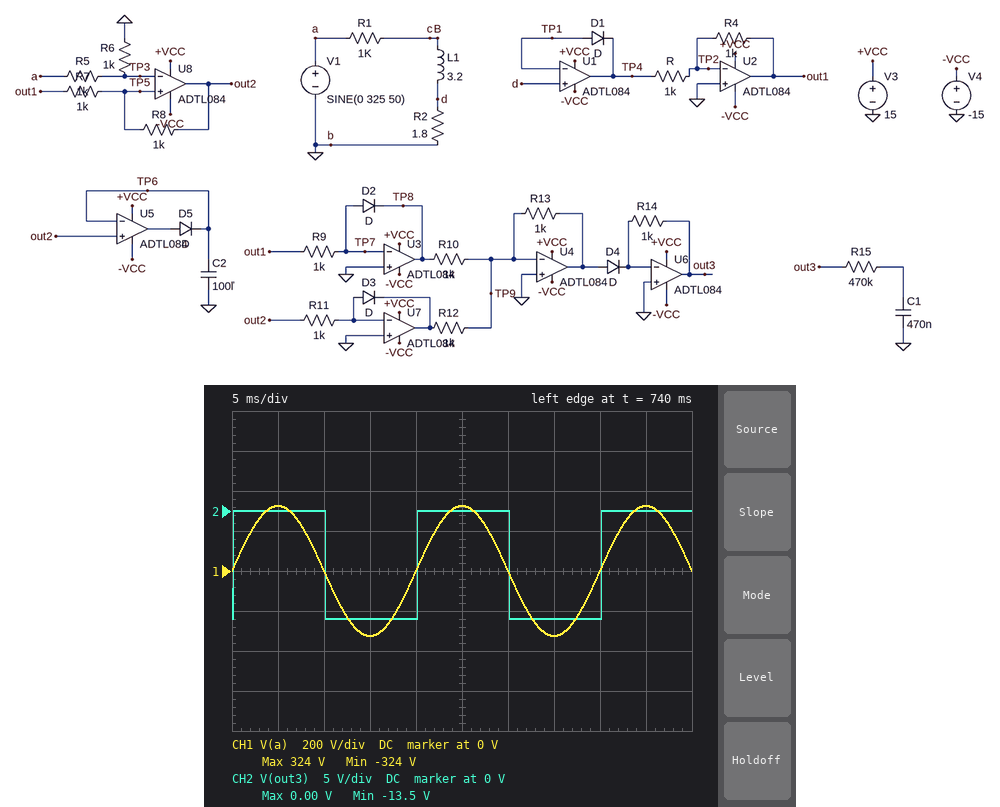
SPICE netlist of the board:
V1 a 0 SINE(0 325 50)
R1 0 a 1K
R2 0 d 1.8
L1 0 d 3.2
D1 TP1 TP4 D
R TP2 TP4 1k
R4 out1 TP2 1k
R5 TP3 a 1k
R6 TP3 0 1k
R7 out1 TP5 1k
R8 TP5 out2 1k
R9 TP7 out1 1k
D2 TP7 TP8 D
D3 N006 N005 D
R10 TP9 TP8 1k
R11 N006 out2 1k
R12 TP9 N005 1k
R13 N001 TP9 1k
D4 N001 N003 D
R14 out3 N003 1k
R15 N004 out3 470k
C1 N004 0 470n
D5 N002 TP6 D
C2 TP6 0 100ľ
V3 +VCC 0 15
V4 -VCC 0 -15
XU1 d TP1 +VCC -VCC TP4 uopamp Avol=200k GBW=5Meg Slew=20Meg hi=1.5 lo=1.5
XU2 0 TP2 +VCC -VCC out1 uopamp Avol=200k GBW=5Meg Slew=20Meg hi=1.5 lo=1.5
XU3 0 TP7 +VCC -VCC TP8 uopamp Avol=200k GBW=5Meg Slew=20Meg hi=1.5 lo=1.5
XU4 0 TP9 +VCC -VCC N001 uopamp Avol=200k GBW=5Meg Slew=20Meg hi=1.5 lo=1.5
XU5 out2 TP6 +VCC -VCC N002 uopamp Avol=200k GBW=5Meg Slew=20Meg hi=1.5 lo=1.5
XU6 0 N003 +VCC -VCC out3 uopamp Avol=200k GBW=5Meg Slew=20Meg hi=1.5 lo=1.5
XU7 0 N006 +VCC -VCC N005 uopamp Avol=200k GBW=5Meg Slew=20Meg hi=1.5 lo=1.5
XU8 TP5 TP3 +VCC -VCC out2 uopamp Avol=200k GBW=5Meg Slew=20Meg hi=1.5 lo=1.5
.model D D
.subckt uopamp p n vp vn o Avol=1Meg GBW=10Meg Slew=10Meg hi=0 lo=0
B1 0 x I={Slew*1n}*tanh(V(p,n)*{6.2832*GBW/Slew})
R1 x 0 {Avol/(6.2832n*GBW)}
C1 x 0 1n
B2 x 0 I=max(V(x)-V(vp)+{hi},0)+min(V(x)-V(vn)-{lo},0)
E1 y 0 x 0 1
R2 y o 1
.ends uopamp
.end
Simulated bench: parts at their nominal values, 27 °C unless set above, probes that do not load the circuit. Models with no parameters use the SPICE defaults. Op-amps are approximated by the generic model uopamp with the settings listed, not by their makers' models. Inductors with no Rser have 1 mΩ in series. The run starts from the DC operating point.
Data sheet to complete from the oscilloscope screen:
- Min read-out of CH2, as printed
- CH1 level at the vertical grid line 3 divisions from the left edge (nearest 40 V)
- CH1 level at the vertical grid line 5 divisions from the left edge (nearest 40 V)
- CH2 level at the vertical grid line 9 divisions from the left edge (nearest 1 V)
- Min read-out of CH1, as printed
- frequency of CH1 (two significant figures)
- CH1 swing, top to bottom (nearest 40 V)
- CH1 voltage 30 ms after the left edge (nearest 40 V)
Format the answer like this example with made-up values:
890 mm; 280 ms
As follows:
-13.5 V; -320 V; 320 V; 0 V; -324 V; 50 Hz; 640 V; 0 V
